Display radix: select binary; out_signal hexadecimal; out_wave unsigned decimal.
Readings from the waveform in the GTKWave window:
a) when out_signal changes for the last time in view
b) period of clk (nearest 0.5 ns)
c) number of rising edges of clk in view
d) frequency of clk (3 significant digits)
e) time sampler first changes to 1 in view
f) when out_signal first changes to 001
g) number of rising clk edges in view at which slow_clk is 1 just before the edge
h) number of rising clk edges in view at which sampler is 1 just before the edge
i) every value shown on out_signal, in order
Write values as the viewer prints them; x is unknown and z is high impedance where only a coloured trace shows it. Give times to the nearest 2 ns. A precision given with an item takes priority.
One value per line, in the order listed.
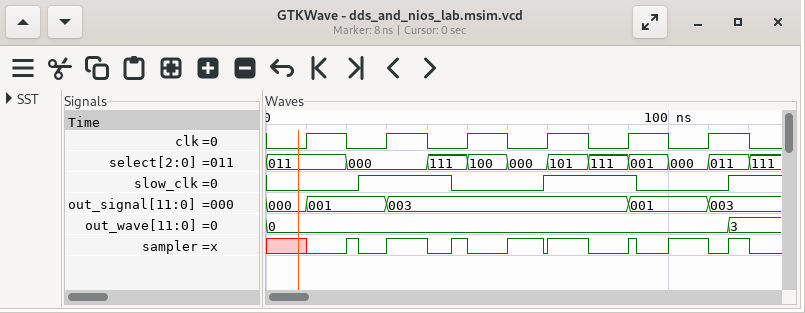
110 ns
20 ns
6
50.0 MHz
20 ns
10 ns
3
2
000, 001, 003, 001, 003
